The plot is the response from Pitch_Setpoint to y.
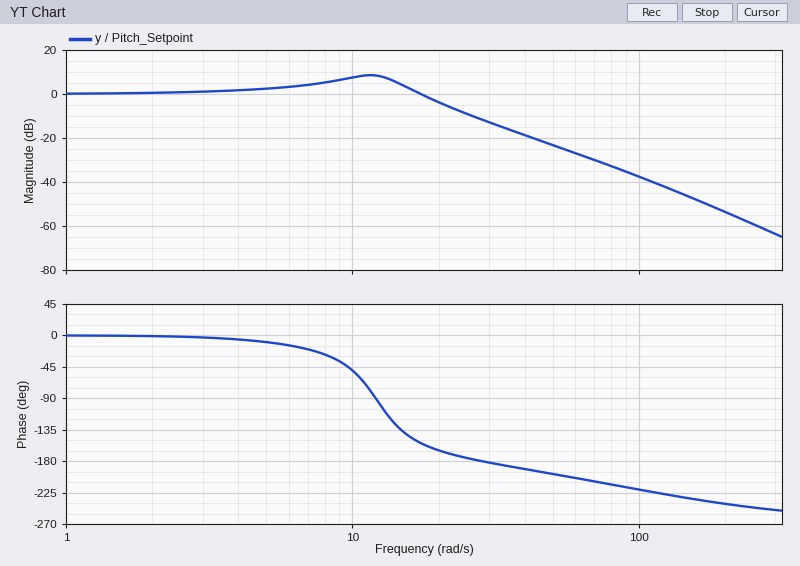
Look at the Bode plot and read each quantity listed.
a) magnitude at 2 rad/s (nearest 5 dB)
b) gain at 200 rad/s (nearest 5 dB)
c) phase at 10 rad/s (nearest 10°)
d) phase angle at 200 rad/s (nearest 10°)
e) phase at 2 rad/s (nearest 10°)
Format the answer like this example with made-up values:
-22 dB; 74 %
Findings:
0 dB; -55 dB; -50°; -240°; 0°
